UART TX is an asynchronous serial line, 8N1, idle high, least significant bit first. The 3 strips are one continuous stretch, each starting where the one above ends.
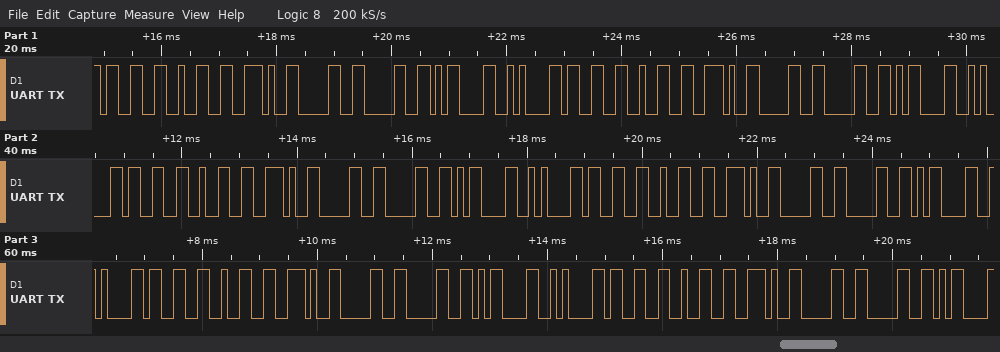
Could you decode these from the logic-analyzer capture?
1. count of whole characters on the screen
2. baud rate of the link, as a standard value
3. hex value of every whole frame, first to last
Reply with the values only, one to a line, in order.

41
9600 baud
33 32 2E 30 30 0D 0A 33 32 2E 30 30 0D 0A 33 32 2E 30 30 0D 0A 33 32 2E 30 30 0D 0A 33 32 2E 30 30 0D 0A 33 32 2E 30 30 0D
